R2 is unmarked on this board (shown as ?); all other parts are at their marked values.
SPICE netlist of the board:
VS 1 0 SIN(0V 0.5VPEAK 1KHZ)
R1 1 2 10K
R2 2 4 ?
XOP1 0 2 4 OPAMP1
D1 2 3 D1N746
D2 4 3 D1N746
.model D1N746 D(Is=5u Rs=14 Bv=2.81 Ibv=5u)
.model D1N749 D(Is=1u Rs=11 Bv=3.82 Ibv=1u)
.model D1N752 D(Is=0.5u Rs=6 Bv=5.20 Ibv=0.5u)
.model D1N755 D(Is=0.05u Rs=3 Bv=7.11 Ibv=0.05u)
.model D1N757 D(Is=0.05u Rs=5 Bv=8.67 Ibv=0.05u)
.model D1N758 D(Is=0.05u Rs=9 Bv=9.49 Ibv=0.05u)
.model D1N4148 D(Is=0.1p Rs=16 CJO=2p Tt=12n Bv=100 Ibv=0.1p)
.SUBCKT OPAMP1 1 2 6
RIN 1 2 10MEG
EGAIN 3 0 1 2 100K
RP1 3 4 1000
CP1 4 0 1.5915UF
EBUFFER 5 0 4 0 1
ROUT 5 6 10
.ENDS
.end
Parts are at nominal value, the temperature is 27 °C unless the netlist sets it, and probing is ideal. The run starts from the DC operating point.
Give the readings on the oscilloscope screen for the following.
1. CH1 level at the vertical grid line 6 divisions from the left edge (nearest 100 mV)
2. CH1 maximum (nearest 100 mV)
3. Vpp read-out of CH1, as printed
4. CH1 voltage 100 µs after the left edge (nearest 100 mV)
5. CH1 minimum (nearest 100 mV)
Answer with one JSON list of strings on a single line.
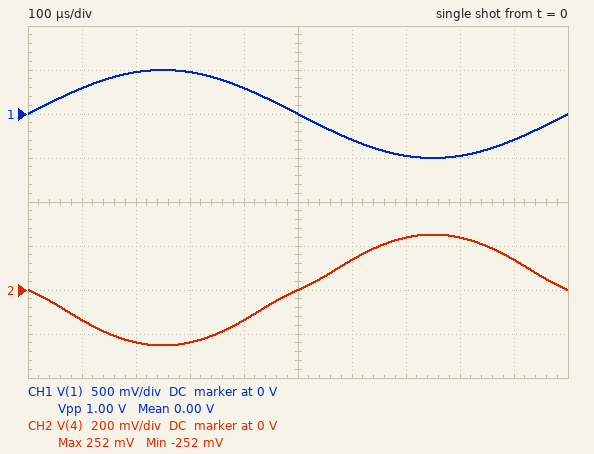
["-300 mV", "500 mV", "1.00 V", "300 mV", "-500 mV"]
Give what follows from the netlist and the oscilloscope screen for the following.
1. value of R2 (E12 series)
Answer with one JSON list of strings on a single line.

["5.6 kΩ"]
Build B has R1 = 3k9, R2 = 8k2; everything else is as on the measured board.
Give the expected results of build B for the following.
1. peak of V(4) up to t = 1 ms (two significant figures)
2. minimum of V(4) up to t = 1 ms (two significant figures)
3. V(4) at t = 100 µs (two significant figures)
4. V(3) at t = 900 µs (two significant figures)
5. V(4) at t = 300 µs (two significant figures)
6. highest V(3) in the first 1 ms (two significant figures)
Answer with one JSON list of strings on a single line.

["1.0 V", "-1.0 V", "-580 mV", "560 mV", "-960 mV", "990 mV"]
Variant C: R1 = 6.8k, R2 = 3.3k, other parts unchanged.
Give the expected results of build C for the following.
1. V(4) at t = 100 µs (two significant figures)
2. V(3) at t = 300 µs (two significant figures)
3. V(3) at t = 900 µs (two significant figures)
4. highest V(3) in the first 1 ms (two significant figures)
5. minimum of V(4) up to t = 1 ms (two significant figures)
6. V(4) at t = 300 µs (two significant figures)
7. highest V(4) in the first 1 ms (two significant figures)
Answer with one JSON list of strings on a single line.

["-130 mV", "-18 mV", "110 mV", "210 mV", "-230 mV", "-210 mV", "230 mV"]
